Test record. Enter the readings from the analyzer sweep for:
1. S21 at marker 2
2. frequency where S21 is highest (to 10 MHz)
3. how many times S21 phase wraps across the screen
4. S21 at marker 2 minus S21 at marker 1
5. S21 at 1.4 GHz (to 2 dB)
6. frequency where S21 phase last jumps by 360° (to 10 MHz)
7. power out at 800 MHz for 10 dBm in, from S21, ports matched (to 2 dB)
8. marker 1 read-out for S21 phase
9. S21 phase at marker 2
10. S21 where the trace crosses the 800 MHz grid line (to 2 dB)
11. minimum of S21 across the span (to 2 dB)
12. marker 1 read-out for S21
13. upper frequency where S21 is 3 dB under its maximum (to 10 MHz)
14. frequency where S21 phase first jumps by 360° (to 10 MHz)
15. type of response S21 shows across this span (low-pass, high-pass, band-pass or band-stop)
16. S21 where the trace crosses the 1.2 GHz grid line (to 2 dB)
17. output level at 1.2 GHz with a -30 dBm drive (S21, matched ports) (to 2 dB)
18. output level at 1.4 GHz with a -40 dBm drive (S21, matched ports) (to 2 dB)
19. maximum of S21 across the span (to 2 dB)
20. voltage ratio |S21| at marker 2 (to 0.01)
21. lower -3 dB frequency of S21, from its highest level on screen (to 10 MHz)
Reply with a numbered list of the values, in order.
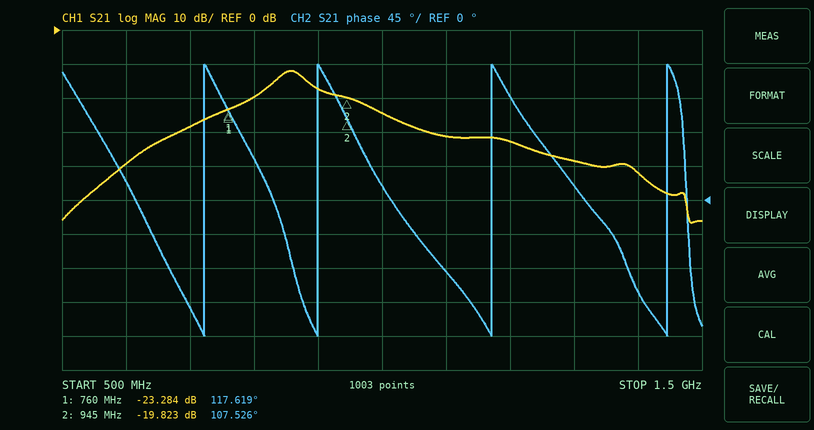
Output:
1. -19.823 dB
2. 860 MHz
3. 4
4. 3.461 dB
5. -42 dB
6. 1.45 GHz
7. -10 dBm
8. 117.619°
9. 107.526°
10. -20 dB
11. -56 dB
12. -23.284 dB
13. 880 MHz
14. 720 MHz
15. band-pass
16. -32 dB
17. -62 dBm
18. -82 dBm
19. -12 dB
20. 0.10
21. 830 MHz
